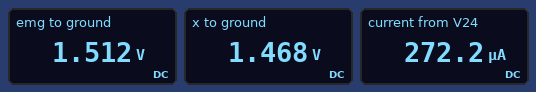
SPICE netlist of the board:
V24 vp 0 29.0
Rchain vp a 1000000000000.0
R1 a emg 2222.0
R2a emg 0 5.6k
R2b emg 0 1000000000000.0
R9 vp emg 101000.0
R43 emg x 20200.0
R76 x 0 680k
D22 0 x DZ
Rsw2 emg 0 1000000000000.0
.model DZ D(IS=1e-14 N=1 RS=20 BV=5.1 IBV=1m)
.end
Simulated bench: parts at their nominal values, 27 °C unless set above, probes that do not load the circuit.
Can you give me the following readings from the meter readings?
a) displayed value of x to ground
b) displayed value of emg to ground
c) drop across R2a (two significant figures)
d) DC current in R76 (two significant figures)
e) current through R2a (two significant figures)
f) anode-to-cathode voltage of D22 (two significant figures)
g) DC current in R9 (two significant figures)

1.468 V
1.512 V
1.5 V
2.2 µA
270 µA
-1.5 V
270 µA
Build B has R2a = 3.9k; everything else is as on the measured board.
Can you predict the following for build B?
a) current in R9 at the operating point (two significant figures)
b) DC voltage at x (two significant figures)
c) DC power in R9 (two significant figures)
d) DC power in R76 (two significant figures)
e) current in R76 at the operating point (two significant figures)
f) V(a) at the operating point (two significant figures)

280 µA
1.0 V
7.7 mW
1.6 µW
1.5 µA
1.1 V
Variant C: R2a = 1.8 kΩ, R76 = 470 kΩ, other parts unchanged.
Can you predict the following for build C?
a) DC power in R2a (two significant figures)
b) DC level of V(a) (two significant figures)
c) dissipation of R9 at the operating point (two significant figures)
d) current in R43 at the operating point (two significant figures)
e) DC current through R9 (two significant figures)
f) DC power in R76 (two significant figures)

140 µW
510 mV
8.0 mW
1.0 µA
280 µA
500 nW
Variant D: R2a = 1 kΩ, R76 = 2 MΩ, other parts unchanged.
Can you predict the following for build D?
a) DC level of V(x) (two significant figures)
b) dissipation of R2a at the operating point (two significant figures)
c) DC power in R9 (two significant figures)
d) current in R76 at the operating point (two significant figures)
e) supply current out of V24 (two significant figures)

280 mV
81 µW
8.2 mW
140 nA
280 µA
